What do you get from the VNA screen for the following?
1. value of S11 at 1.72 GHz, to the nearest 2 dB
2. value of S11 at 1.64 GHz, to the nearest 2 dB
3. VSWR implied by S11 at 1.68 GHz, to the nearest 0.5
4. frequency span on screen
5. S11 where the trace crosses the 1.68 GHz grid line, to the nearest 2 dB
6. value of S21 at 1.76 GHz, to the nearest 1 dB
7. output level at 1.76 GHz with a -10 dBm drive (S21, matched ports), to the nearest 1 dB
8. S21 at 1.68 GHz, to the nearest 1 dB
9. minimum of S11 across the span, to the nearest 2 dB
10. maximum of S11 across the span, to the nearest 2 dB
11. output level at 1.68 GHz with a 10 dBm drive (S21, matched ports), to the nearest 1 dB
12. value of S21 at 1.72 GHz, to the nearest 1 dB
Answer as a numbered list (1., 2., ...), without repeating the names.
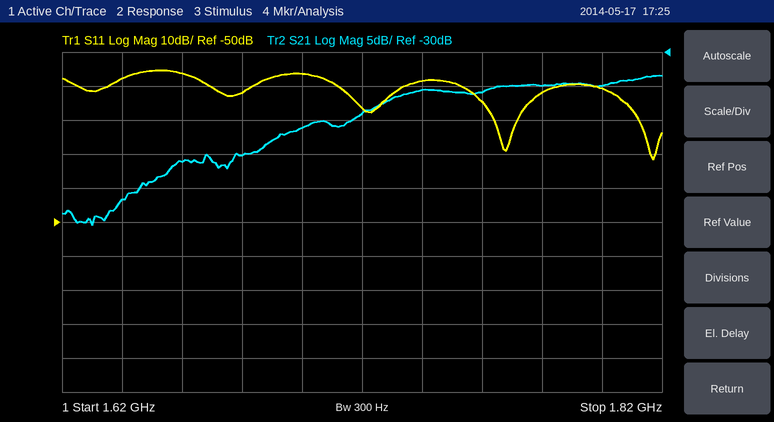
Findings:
1. -16 dB
2. -8 dB
3. 1.5
4. 200 MHz
5. -12 dB
6. -36 dB
7. -46 dBm
8. -45 dB
9. -32 dB
10. -6 dB
11. -35 dBm
12. -39 dB
